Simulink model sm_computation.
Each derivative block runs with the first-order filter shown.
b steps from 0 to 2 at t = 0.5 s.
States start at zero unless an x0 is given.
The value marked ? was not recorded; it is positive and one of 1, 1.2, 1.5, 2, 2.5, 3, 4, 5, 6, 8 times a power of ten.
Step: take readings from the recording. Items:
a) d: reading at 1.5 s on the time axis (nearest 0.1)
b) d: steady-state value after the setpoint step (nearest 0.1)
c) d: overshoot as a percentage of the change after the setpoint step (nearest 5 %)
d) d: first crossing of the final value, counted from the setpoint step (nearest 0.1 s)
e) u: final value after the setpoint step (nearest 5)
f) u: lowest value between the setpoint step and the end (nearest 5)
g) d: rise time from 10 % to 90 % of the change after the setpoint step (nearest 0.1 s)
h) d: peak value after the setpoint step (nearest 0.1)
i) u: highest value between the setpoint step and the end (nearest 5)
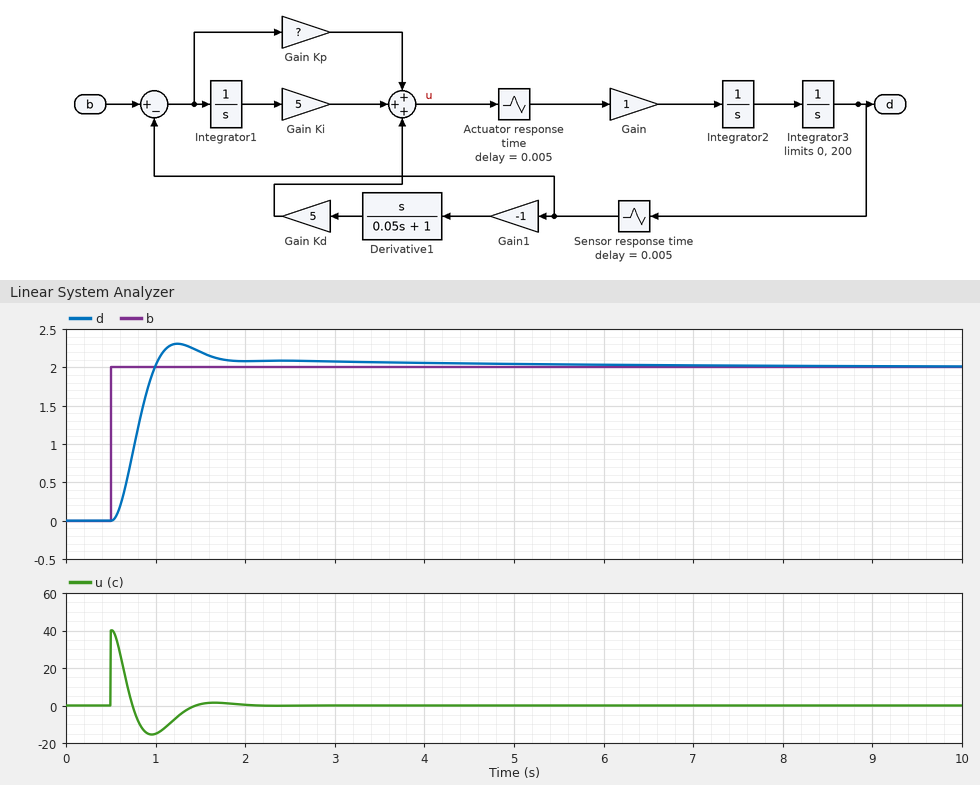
2.2
2.0
15 %
0.5 s
0
-15
0.3 s
2.3
40
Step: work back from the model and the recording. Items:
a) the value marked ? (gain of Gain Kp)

20
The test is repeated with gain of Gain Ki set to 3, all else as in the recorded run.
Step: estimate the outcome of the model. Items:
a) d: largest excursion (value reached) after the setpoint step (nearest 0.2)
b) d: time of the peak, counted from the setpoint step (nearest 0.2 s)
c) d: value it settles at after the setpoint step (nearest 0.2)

2.2
0.8 s
2.0
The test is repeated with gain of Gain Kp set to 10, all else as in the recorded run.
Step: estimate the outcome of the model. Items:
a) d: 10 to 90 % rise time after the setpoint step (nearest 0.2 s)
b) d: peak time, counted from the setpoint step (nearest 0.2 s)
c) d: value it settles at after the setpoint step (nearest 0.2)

0.6 s
1.6 s
2.0
